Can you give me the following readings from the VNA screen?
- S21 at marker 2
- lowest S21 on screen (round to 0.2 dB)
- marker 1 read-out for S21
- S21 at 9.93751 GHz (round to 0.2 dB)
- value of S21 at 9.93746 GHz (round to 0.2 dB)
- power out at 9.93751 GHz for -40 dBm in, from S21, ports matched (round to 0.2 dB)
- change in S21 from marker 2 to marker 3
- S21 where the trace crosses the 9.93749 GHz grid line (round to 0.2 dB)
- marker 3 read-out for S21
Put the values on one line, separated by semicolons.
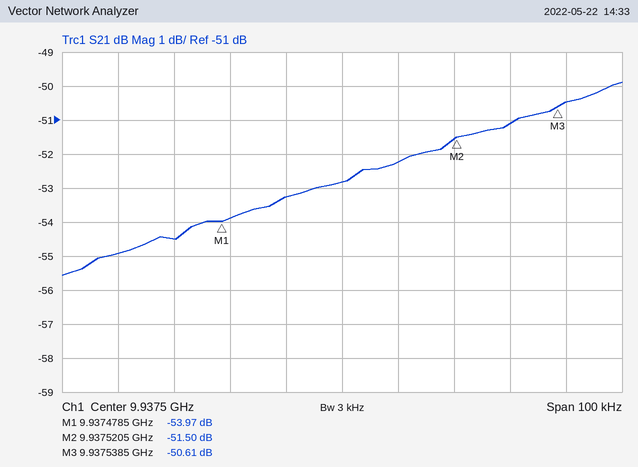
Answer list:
-51.50 dB; -55.6 dB; -53.97 dB; -52.2 dB; -55.0 dB; -92.2 dBm; 0.89 dB; -53.2 dB; -50.61 dB
